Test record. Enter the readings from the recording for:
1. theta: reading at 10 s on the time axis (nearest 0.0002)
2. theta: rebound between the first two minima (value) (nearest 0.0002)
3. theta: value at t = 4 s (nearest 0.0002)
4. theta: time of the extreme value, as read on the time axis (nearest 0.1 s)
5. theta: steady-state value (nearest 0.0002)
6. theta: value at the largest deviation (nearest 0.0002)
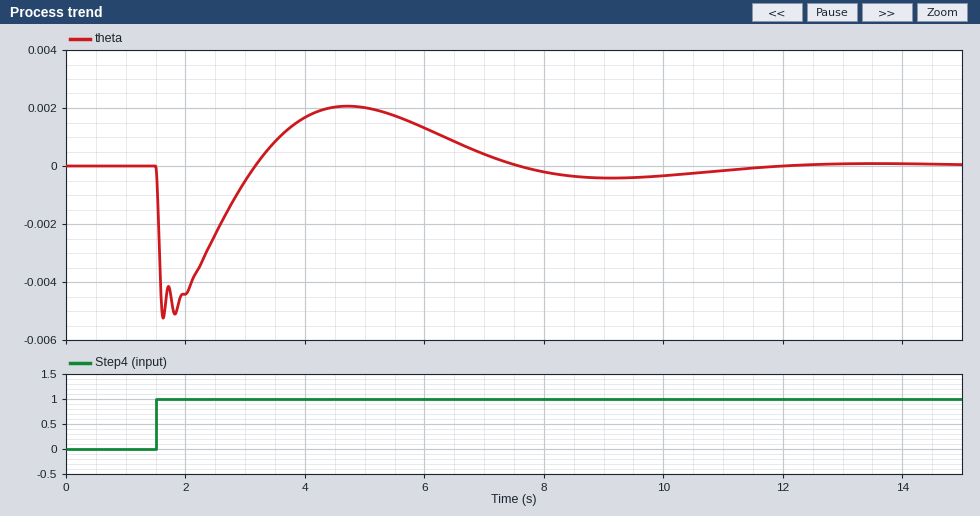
-0.0004
-0.0042
0.0016
1.6 s
0.0000
-0.0052
